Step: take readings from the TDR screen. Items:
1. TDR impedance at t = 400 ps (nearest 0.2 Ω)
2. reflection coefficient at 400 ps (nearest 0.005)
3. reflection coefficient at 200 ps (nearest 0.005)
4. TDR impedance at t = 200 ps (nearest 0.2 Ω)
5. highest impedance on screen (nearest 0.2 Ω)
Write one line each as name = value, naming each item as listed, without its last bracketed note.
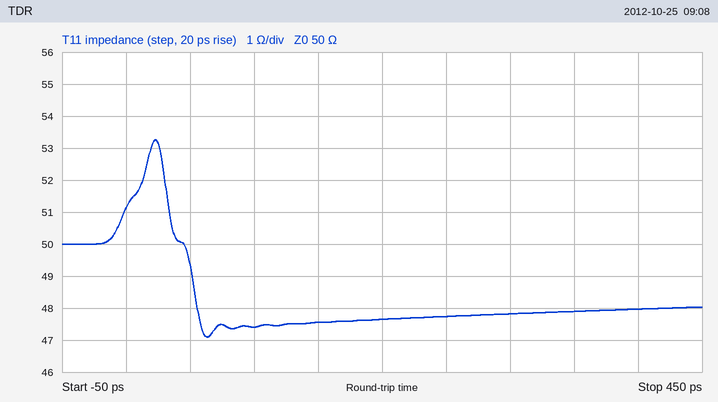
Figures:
TDR impedance at t = 400 ps = 48.0 Ω
reflection coefficient at 400 ps = -0.020
reflection coefficient at 200 ps = -0.025
TDR impedance at t = 200 ps = 47.6 Ω
highest impedance on screen = 53.2 Ω
